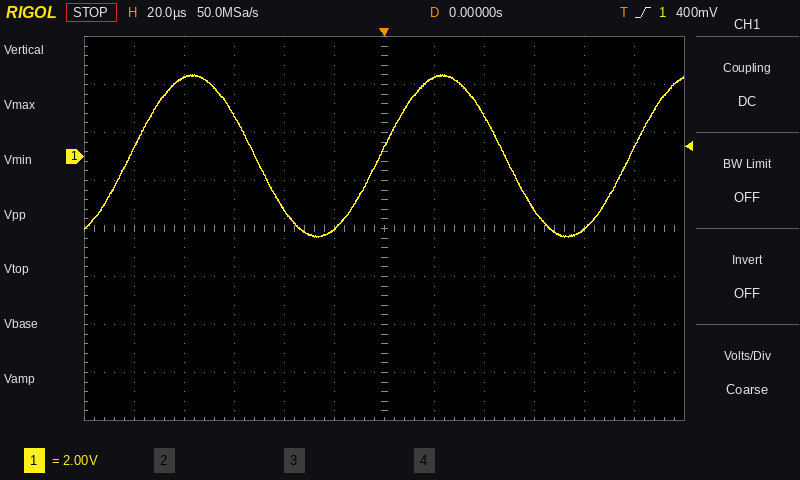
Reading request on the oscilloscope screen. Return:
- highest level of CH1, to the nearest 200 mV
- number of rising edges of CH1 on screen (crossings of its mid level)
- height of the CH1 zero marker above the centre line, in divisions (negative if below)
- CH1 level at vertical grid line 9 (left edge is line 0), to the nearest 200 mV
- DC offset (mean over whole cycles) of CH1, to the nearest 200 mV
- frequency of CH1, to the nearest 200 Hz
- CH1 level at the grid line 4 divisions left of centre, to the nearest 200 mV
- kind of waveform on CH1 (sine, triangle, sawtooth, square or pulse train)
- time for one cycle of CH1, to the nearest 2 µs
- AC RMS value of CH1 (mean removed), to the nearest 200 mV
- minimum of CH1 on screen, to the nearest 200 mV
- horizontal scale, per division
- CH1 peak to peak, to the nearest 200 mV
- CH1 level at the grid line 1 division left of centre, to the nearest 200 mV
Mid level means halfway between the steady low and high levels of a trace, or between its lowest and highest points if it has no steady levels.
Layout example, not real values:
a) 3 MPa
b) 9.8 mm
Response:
a) 3.4 V
b) 3
c) +1.5 div
d) -2.2 V
e) 0.0 V
f) 10.0 kHz
g) 3.2 V
h) sine
i) 100 µs
j) 2.4 V
k) -3.4 V
l) 20 µs
m) 6.8 V
n) -3.0 V
